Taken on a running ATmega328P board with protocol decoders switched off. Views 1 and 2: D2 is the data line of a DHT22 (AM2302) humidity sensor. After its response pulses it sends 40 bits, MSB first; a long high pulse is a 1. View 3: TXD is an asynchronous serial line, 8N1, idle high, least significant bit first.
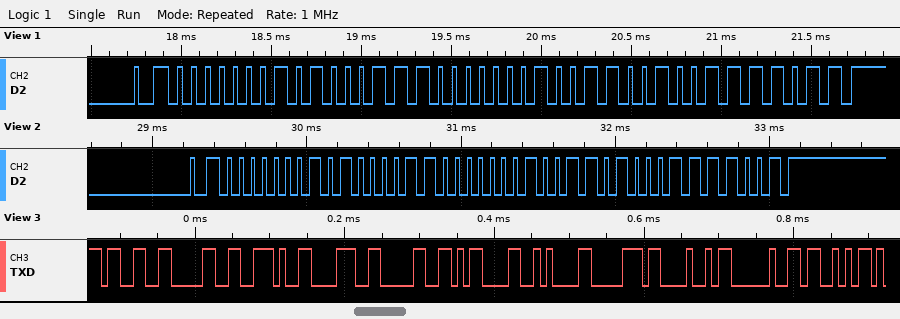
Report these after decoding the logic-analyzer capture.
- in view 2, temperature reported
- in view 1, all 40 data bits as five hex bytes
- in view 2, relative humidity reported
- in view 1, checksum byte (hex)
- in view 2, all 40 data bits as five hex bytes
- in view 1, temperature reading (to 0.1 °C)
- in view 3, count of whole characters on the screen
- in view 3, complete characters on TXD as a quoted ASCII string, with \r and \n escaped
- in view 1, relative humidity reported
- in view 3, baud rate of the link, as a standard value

30.8 °C
01 47 01 32 7B
32.3 %
0x7B
01 43 01 34 79
30.6 °C
11
"30.80\r\npH S"
32.7 %
115200 baud
